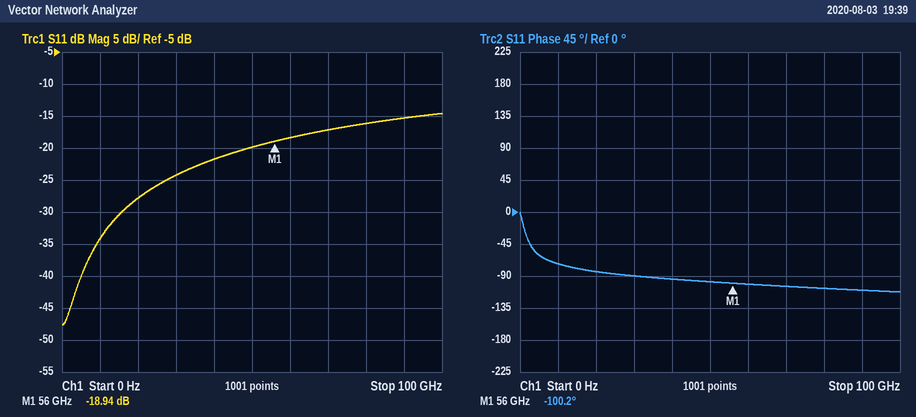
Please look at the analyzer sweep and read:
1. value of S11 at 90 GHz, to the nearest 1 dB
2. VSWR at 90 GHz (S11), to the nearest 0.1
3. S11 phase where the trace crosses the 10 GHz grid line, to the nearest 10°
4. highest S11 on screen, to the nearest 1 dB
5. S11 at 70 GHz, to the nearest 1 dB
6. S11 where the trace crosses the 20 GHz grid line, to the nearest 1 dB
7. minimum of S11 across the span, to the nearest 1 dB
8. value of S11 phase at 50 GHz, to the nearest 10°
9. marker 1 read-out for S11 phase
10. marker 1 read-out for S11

-15 dB
1.4
-70°
-15 dB
-17 dB
-28 dB
-48 dB
-100°
-100.2°
-18.94 dB
